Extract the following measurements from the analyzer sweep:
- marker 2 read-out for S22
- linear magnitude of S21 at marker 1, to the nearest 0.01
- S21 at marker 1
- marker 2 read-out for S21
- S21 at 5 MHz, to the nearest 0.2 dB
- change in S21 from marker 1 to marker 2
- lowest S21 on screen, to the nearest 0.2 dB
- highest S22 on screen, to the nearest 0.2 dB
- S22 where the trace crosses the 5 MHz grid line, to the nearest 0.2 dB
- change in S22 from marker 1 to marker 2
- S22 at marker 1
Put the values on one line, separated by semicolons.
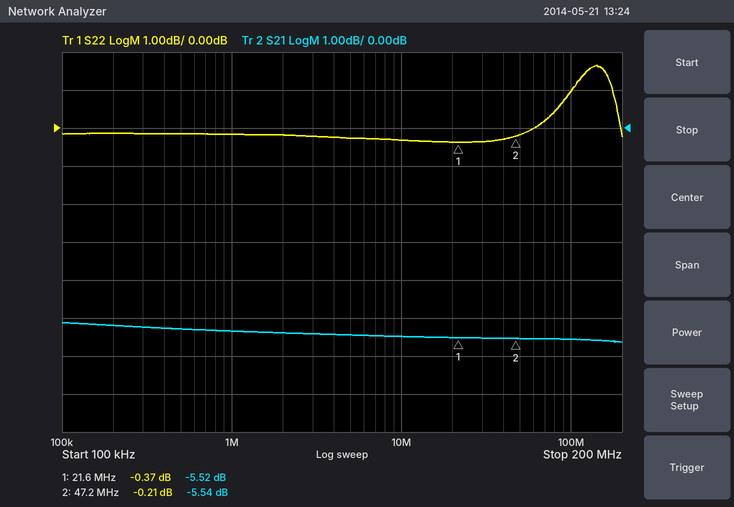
-0.21 dB; 0.53; -5.52 dB; -5.54 dB; -5.4 dB; -0.02 dB; -5.6 dB; 1.6 dB; -0.2 dB; 0.16 dB; -0.37 dB
